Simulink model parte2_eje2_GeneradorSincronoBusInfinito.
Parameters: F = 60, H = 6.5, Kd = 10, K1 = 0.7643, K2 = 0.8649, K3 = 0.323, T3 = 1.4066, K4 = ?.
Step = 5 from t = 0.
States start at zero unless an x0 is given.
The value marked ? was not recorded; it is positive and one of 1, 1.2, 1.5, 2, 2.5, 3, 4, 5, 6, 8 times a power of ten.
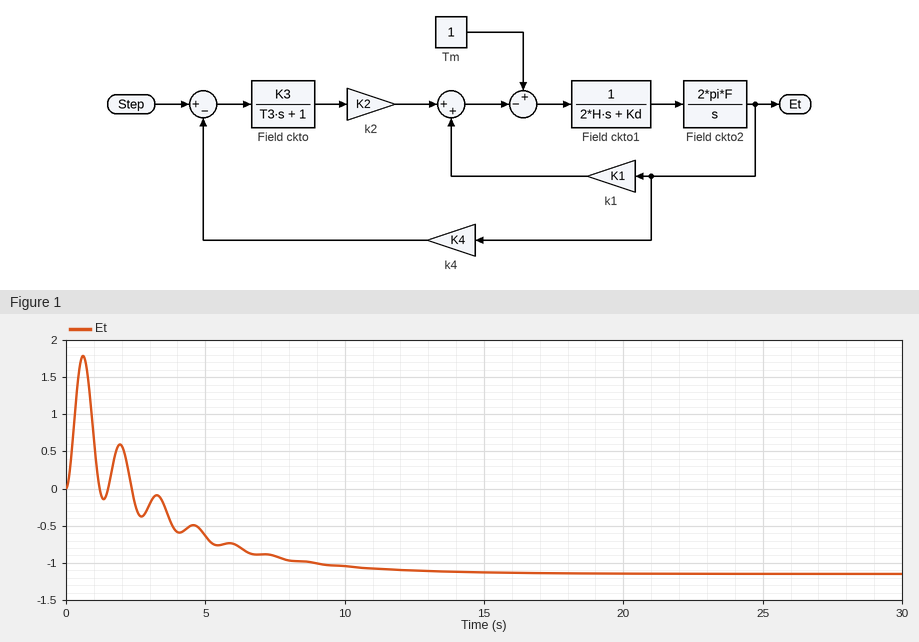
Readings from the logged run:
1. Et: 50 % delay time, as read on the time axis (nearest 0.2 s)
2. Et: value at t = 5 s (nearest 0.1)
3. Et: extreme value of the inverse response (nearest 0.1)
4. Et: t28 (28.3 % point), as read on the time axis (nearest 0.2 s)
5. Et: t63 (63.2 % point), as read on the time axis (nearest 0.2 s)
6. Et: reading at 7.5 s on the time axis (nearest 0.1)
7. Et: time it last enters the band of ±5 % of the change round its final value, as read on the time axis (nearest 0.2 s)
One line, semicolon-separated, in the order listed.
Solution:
4.0 s; -0.6; 1.8; 2.6 s; 5.2 s; -0.9; 11.8 s
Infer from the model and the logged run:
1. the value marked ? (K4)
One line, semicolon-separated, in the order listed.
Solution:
1.5
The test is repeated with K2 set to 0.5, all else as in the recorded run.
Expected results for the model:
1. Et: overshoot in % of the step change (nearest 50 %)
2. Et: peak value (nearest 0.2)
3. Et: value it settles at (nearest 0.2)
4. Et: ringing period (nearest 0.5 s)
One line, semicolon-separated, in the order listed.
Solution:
450 %; 2.0; 0.4; 1.5 s
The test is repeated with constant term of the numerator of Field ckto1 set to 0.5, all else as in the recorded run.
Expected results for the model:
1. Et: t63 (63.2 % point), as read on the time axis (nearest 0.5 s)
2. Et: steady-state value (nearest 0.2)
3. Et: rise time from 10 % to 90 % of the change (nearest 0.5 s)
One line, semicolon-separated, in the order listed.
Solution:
5.5 s; -1.2; 8.0 s
